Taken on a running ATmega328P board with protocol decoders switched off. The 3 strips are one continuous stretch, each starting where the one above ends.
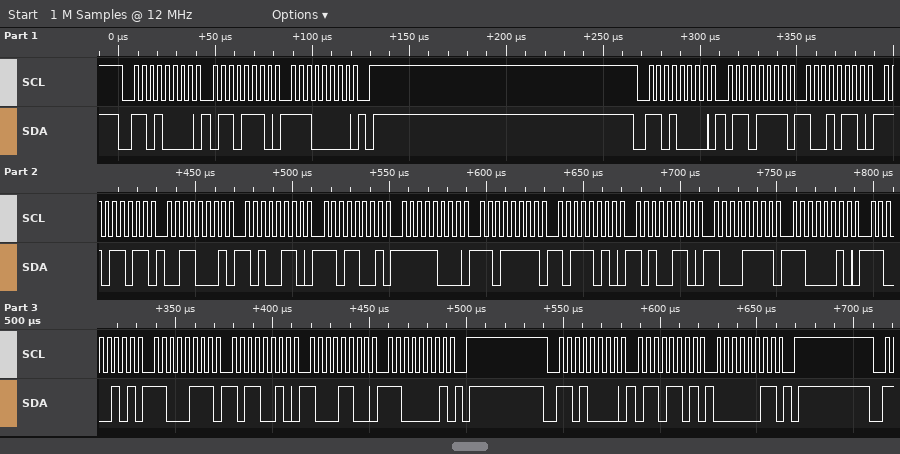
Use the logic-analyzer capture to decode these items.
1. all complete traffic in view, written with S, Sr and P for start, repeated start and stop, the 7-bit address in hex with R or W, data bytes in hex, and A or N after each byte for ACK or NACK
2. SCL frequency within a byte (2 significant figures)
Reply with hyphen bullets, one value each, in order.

- S 68W A 6E A E0 A P S 68W A 6F A 96 A DB A 31 A A6 A D9 A F8 A DF A BA A A6 A 8F A C2 A C5 A C7 A B2 A 8C A C1 A P S 68W A 6D A 03 A P
- 250 kHz
